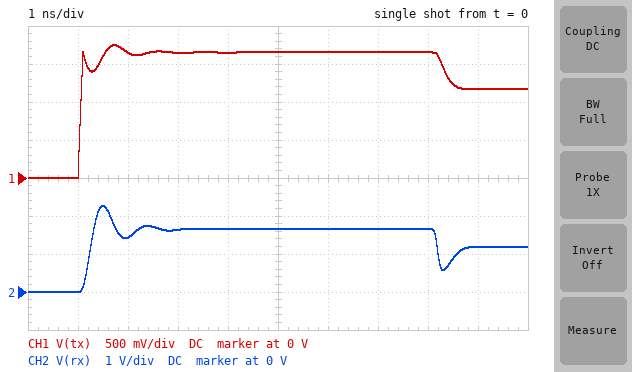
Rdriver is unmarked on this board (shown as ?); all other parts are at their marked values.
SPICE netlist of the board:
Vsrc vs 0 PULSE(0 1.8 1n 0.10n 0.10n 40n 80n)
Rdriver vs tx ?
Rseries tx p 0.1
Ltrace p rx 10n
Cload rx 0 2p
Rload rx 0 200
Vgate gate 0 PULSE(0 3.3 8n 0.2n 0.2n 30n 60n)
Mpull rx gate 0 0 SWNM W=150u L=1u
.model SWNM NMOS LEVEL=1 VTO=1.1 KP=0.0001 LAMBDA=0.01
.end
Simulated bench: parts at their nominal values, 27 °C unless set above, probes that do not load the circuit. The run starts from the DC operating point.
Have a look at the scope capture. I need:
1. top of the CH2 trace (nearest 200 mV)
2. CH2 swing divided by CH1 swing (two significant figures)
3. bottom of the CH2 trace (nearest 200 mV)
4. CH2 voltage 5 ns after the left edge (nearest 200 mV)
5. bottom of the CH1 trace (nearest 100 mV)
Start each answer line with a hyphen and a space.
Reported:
- 2.2 V
- 1.3
- 0 V
- 1.6 V
- 0 V
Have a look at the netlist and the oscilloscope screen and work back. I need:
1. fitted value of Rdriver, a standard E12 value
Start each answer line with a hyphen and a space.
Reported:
- 18 Ω
